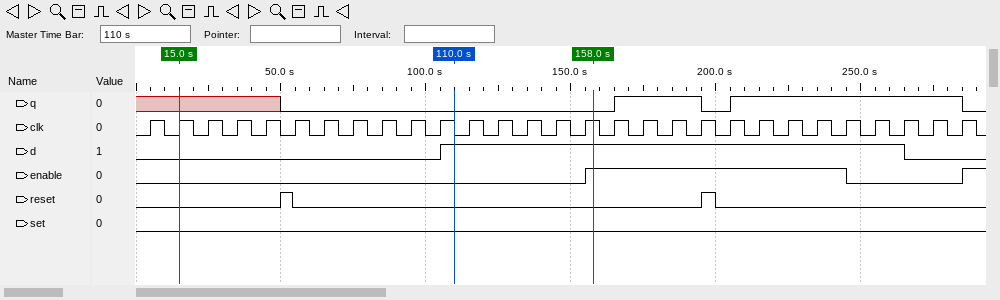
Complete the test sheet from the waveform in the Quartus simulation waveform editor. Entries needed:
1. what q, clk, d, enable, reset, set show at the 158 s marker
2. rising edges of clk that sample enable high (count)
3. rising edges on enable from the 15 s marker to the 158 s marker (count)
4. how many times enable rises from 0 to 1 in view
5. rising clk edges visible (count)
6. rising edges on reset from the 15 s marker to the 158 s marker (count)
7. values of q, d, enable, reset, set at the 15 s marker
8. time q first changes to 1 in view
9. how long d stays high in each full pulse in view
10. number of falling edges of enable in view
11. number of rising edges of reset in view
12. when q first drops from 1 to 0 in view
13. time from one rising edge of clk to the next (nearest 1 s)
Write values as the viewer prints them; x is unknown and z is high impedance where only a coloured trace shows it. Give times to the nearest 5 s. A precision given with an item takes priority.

q=0, clk=1, d=1, enable=1, reset=0, set=0
9
1
2
29
1
q=x, d=0, enable=0, reset=0, set=0
165 s
160 s
1
2
195 s
10 s
